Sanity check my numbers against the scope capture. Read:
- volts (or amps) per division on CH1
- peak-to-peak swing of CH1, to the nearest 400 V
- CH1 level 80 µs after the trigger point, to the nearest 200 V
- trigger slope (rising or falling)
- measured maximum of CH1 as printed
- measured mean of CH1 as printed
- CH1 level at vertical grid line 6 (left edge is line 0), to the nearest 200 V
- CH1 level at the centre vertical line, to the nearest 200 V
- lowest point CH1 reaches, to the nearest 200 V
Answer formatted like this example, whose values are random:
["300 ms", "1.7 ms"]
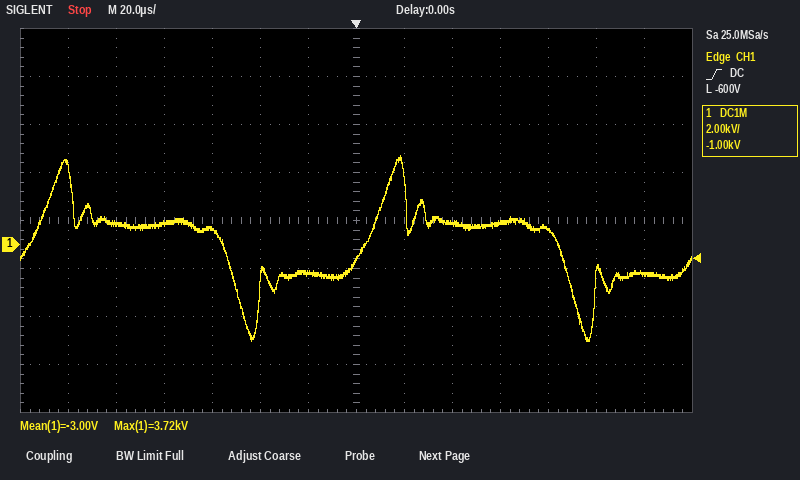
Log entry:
["2 kV", "7.6 kV", "600 V", "rising", "3.72 kV", "-3.00 V", "-1.2 kV", "-600 V", "-4.0 kV"]
